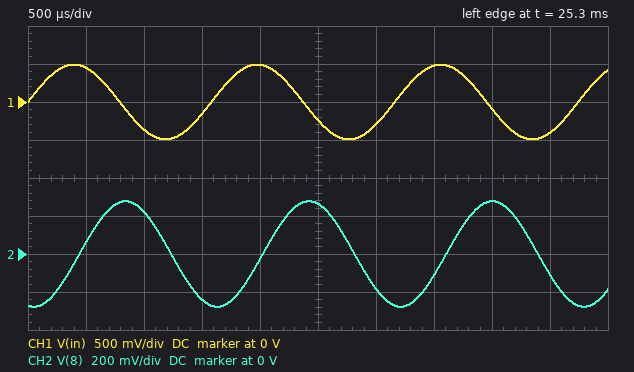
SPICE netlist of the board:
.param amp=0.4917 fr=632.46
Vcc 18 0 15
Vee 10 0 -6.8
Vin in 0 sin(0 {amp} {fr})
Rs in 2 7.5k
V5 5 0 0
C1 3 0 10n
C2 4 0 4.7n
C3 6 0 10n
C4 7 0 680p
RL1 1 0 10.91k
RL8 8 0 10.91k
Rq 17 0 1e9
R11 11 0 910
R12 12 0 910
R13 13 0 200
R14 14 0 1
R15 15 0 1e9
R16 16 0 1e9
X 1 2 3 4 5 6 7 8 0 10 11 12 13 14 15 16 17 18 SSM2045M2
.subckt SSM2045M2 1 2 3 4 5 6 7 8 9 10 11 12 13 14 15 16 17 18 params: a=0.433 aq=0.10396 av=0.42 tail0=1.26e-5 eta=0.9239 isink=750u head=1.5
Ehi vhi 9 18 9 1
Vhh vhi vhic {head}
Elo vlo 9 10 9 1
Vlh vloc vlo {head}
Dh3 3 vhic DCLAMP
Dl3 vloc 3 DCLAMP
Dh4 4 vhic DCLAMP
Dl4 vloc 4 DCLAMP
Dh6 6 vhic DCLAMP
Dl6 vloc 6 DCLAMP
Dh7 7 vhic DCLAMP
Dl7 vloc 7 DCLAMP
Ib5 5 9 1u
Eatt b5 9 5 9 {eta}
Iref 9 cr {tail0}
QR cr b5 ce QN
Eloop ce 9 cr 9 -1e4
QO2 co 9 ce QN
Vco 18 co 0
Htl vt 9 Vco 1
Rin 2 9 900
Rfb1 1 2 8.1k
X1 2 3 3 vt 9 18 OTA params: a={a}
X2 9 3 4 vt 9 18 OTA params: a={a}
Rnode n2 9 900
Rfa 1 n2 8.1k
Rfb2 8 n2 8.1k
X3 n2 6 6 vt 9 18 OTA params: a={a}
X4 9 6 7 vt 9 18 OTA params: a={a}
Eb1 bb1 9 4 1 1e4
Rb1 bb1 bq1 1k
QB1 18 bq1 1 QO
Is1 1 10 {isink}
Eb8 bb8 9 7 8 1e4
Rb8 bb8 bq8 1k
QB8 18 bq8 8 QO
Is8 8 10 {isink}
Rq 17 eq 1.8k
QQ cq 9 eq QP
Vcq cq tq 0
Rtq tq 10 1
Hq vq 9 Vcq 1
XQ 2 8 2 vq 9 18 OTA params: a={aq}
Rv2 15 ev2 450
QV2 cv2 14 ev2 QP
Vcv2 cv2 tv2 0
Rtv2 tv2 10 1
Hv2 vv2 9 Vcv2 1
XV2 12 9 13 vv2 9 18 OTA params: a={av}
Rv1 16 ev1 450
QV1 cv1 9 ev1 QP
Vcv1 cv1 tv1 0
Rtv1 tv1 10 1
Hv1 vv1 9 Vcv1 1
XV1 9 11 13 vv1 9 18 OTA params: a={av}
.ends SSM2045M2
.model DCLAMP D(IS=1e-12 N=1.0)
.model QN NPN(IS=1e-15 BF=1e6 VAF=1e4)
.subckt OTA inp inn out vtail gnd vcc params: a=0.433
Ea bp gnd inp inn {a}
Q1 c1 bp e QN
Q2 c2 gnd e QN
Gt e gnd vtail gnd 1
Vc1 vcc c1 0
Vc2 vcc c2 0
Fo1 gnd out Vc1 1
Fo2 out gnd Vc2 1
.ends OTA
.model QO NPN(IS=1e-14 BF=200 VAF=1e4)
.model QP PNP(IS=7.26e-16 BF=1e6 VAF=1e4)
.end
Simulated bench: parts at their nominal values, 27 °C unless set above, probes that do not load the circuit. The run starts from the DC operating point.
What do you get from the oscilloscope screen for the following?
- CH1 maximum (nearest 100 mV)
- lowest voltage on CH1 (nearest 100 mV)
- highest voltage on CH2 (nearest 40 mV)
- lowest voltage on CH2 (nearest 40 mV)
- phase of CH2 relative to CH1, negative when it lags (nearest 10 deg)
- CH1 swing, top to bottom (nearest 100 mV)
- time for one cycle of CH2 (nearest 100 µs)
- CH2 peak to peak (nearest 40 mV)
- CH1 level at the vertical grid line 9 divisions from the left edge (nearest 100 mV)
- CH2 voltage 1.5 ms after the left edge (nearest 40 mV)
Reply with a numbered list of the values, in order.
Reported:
1. 500 mV
2. -500 mV
3. 280 mV
4. -280 mV
5. -100 deg
6. 1.0 V
7. 1.6 ms
8. 560 mV
9. -400 mV
10. -240 mV
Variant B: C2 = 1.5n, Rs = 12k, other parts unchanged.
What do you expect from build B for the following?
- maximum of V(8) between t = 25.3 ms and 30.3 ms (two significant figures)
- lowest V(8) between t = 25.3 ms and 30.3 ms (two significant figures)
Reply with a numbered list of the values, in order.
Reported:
1. 360 mV
2. -360 mV
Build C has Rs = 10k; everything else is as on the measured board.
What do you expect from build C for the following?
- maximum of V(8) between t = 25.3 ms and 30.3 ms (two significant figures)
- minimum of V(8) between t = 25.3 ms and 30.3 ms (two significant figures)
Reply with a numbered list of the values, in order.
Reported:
1. 220 mV
2. -220 mV
